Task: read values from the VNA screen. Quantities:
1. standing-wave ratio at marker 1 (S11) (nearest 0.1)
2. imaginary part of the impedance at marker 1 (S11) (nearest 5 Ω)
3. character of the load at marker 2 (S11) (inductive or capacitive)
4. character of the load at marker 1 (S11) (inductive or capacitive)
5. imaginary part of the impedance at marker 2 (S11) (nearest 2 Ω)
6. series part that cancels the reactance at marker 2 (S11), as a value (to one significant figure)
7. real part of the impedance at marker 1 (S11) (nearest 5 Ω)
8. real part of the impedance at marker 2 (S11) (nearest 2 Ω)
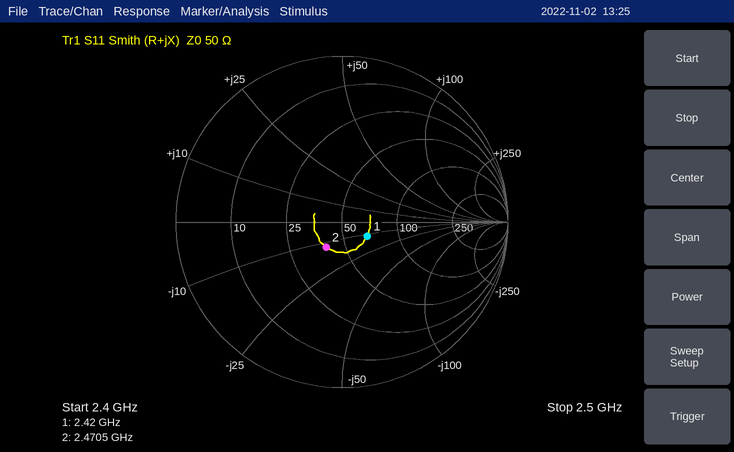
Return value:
1.4
-10 Ω
capacitive
capacitive
-12 Ω
800 pH
65 Ω
40 Ω
